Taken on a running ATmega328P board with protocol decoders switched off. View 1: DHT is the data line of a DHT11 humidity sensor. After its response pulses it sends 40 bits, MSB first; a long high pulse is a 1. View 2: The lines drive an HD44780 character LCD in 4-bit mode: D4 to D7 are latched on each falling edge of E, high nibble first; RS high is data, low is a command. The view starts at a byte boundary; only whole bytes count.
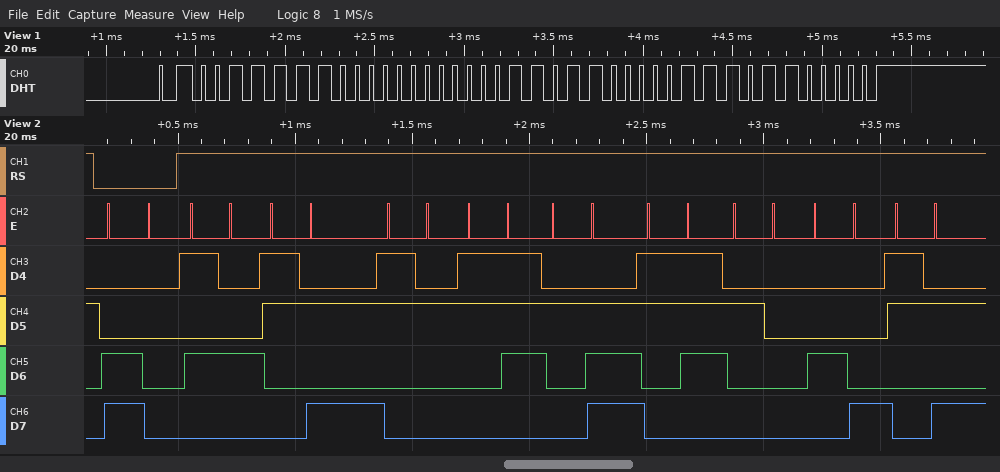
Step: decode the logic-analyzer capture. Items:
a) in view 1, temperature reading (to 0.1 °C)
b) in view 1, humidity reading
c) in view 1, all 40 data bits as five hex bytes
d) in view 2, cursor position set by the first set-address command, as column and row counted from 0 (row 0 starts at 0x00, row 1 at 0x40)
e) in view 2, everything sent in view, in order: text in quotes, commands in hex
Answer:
27.7 °C
62 %
3E 00 1B 07 60
column 0, row 1
0xC0 "T:27.7 H:"
